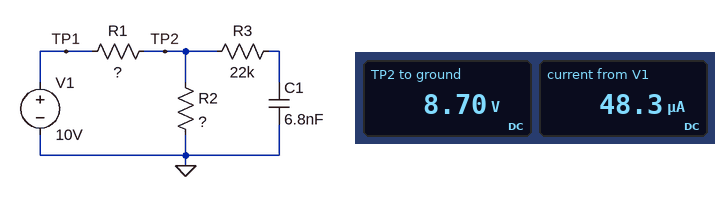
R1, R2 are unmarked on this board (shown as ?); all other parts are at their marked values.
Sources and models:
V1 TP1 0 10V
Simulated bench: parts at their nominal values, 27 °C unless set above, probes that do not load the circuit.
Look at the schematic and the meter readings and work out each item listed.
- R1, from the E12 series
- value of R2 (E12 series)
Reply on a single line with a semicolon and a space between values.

27 kΩ; 180 kΩ
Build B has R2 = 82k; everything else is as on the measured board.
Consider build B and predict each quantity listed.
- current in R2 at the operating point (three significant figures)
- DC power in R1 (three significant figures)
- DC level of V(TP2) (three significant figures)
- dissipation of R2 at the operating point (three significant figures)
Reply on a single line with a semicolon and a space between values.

91.7 µA; 227 µW; 7.52 V; 690 µW
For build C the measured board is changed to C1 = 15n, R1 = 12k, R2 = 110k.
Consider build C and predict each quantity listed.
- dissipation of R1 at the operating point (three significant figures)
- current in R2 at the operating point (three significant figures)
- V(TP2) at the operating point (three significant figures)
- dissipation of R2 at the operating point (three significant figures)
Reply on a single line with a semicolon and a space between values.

80.6 µW; 82.0 µA; 9.02 V; 739 µW
